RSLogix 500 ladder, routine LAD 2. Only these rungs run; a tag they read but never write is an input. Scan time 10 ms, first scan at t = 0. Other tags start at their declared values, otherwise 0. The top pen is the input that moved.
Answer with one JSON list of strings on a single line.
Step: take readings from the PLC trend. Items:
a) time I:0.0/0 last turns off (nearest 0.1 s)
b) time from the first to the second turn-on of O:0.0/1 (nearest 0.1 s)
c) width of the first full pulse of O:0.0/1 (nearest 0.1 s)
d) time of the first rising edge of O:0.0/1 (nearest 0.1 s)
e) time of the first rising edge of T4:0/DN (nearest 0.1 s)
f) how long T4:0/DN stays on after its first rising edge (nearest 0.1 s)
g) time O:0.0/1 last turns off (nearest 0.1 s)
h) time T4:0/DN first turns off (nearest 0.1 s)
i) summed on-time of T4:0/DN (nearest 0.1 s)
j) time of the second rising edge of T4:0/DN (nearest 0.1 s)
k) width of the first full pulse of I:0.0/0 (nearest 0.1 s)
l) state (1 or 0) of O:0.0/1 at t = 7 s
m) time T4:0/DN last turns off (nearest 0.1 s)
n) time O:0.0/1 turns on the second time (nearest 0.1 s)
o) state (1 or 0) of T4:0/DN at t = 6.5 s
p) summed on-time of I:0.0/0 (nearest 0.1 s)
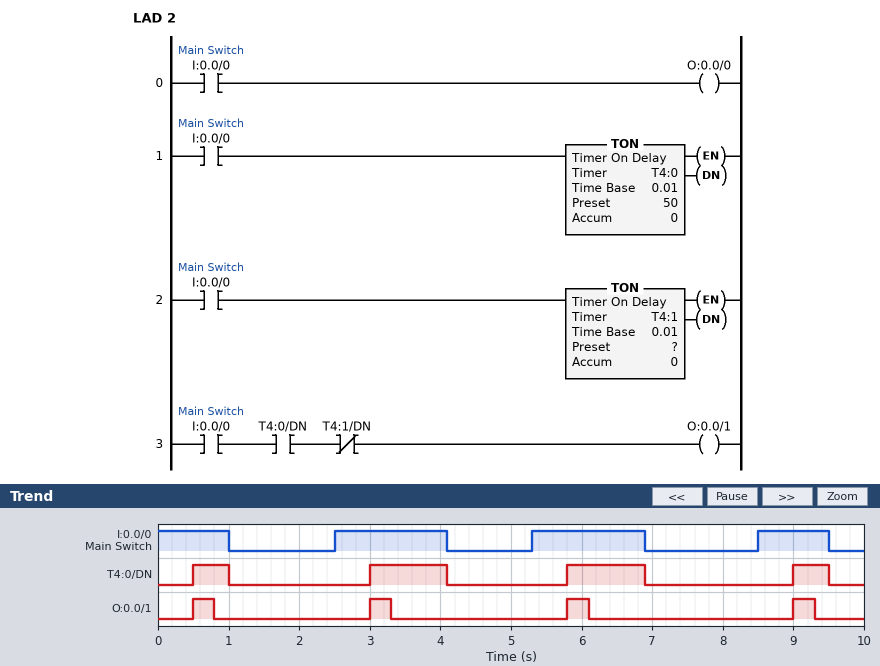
["9.5 s", "2.5 s", "0.3 s", "0.5 s", "0.5 s", "0.5 s", "9.3 s", "1.0 s", "3.2 s", "3.0 s", "1.6 s", "0", "9.5 s", "3.0 s", "1", "5.2 s"]
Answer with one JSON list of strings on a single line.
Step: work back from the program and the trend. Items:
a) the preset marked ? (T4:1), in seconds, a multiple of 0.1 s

["0.8 s"]
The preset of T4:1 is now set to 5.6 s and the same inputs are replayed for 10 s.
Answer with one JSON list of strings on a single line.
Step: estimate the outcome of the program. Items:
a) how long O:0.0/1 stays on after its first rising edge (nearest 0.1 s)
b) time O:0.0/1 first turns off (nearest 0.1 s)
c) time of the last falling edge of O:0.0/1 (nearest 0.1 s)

["0.5 s", "1.0 s", "9.5 s"]
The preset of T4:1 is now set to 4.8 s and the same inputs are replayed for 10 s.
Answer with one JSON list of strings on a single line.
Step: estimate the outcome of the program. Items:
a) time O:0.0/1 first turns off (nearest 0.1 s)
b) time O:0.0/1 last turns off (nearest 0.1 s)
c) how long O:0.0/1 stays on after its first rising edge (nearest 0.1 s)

["1.0 s", "9.5 s", "0.5 s"]
